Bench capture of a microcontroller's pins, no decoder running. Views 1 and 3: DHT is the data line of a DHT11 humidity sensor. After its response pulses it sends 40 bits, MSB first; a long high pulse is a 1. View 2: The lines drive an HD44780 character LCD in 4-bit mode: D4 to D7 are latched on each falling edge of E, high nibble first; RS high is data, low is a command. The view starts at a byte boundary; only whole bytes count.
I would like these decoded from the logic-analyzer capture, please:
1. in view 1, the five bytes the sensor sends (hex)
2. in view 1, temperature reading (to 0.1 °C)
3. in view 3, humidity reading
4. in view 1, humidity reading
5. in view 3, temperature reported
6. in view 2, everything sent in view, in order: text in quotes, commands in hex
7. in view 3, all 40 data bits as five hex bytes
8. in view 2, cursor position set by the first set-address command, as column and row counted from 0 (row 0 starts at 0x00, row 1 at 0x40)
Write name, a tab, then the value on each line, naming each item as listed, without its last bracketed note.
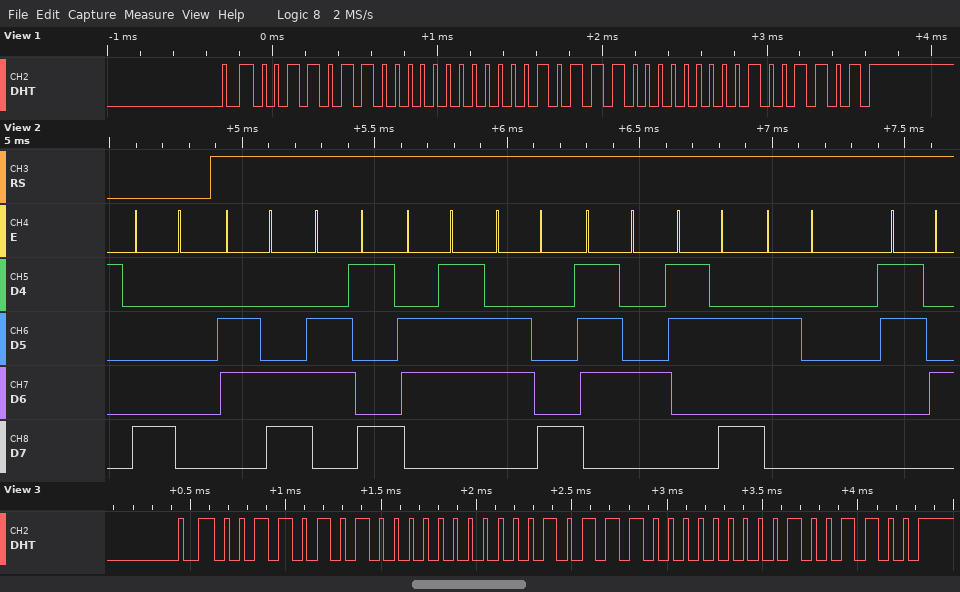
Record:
in view 1, the five bytes the sensor sends	36 00 17 00 4D
in view 1, temperature reading	23.0 °C
in view 3, humidity reading	53 %
in view 1, humidity reading	54 %
in view 3, temperature reported	23.0 °C
in view 2, everything sent in view, in order: text in quotes, commands in hex	0x80 "light: 4"
in view 3, all 40 data bits as five hex bytes	35 00 17 00 4C
in view 2, cursor position set by the first set-address command, as column and row counted from 0	column 0, row 0
